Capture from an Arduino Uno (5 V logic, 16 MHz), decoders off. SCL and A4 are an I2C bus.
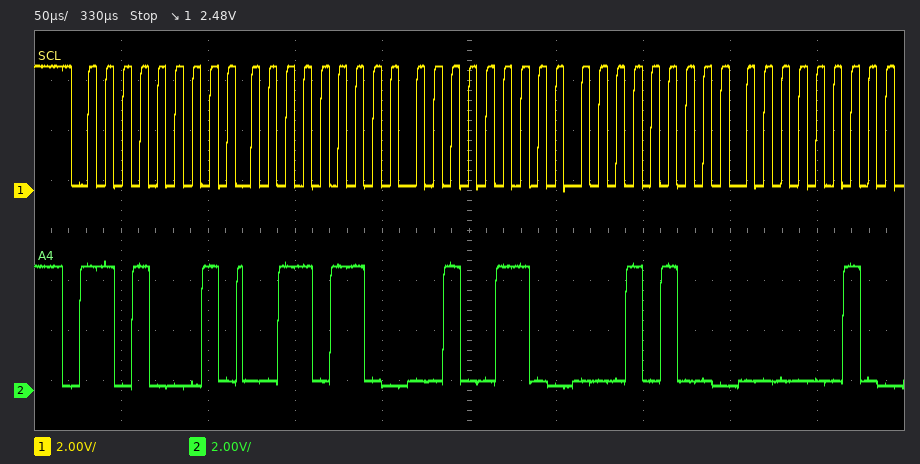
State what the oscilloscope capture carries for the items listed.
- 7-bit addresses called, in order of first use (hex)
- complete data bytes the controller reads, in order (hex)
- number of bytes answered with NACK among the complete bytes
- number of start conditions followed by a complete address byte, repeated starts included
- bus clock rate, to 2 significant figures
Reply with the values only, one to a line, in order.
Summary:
0x68
36 26 14 02
0
1
100 kHz
